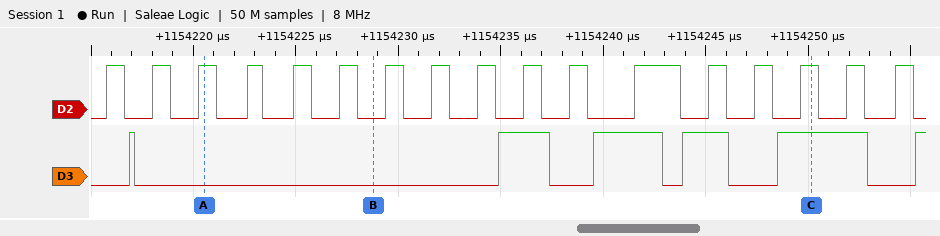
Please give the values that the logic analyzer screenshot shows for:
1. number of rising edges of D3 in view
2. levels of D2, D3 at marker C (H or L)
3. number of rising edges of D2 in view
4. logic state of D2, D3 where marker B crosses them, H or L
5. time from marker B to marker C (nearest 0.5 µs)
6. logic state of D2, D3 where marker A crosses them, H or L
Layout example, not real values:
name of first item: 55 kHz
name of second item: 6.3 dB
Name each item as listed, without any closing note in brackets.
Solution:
number of rising edges of D3 in view: 6
levels of D2, D3 at marker C: D2=H, D3=H
number of rising edges of D2 in view: 17
logic state of D2, D3 where marker B crosses them, H or L: D2=L, D3=L
time from marker B to marker C: 21.5 µs
logic state of D2, D3 where marker A crosses them, H or L: D2=H, D3=L
